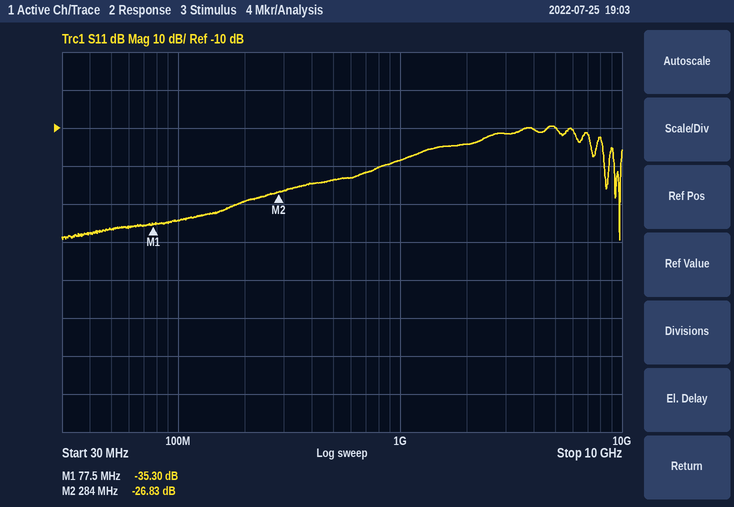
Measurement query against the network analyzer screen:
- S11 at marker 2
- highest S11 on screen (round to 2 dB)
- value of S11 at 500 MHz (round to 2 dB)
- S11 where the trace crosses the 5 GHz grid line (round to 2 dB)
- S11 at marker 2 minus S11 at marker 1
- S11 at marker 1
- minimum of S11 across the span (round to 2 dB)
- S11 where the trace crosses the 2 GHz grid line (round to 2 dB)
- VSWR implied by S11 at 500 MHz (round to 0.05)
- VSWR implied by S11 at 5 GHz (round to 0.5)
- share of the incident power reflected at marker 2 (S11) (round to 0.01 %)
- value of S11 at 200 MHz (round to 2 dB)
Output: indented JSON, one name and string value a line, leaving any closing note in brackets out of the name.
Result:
{
  "S11 at marker 2": "-26.83 dB",
  "highest S11 on screen": "-10 dB",
  "value of S11 at 500 MHz": "-24 dB",
  "S11 where the trace crosses the 5 GHz grid line": "-10 dB",
  "S11 at marker 2 minus S11 at marker 1": "8.47 dB",
  "S11 at marker 1": "-35.30 dB",
  "minimum of S11 across the span": "-40 dB",
  "S11 where the trace crosses the 2 GHz grid line": "-14 dB",
  "VSWR implied by S11 at 500 MHz": "1.15",
  "VSWR implied by S11 at 5 GHz": "2.0",
  "share of the incident power reflected at marker 2 (S11)": "0.21 %",
  "value of S11 at 200 MHz": "-30 dB"
}
